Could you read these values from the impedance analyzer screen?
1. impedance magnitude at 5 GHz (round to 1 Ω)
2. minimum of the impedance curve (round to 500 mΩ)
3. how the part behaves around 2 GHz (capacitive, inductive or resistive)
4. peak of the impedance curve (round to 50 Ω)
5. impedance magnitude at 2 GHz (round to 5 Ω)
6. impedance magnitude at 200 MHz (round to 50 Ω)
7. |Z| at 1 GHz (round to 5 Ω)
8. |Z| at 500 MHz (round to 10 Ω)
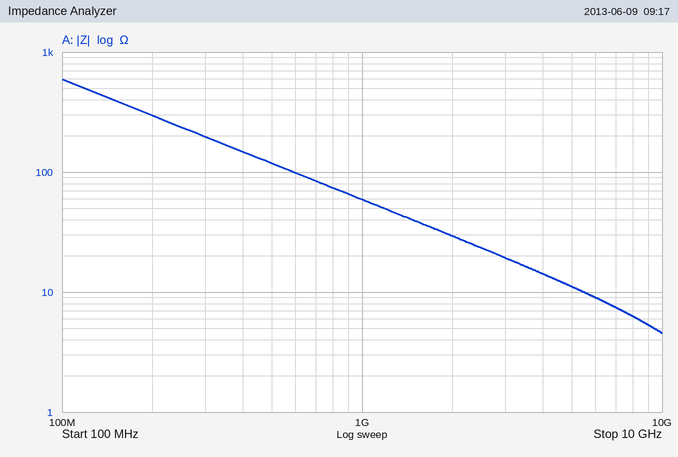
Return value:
11 Ω
4.5 Ω
capacitive
600 Ω
30 Ω
300 Ω
60 Ω
120 Ω
